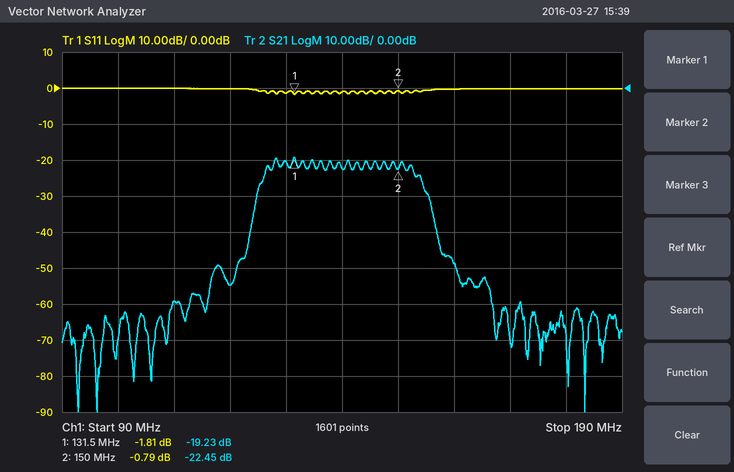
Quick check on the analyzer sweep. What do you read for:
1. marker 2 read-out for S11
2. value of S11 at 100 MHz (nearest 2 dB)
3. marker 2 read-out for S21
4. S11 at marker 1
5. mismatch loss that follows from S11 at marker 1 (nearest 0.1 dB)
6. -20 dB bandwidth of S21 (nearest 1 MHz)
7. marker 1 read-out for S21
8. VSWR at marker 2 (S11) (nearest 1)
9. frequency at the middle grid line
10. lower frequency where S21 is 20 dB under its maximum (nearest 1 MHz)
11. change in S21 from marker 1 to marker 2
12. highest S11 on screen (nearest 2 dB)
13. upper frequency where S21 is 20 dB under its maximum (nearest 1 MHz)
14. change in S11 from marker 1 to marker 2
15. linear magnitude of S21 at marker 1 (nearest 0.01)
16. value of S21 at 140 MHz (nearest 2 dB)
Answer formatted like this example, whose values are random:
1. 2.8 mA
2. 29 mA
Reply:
1. -0.79 dB
2. 0 dB
3. -22.45 dB
4. -1.81 dB
5. 4.7 dB
6. 33 MHz
7. -19.23 dB
8. 22
9. 140 MHz
10. 124 MHz
11. -3.22 dB
12. 0 dB
13. 157 MHz
14. 1.02 dB
15. 0.11
16. -22 dB
